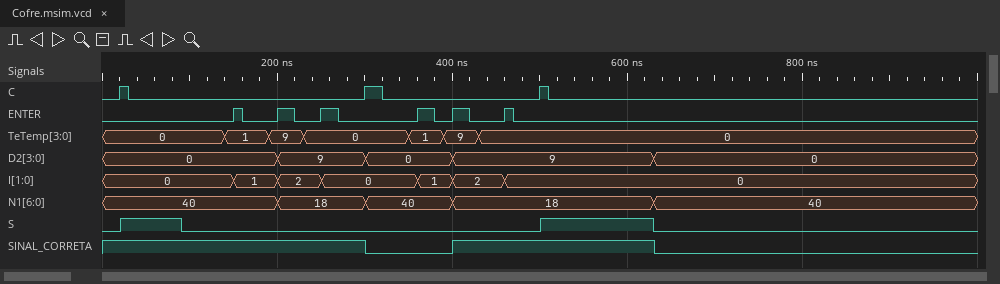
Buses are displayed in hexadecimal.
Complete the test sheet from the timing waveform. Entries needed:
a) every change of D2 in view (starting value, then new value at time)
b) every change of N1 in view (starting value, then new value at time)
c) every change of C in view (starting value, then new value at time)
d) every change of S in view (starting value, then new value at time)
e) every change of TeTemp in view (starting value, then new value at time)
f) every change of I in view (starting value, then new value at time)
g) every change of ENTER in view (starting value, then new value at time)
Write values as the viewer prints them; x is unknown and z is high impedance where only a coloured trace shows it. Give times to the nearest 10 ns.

0, 9 at 200 ns, 0 at 300 ns, 9 at 400 ns, 0 at 630 ns
40, 18 at 200 ns, 40 at 300 ns, 18 at 400 ns, 40 at 630 ns
0, 1 at 20 ns, 0 at 30 ns, 1 at 300 ns, 0 at 320 ns, 1 at 500 ns, 0 at 510 ns
0, 1 at 20 ns, 0 at 90 ns, 1 at 500 ns, 0 at 630 ns
0, 1 at 140 ns, 9 at 190 ns, 0 at 230 ns, 1 at 350 ns, 9 at 390 ns, 0 at 430 ns
0, 1 at 150 ns, 2 at 200 ns, 0 at 250 ns, 1 at 360 ns, 2 at 400 ns, 0 at 460 ns
0, 1 at 150 ns, 0 at 160 ns, 1 at 200 ns, 0 at 220 ns, 1 at 250 ns, 0 at 270 ns, 1 at 360 ns, 0 at 380 ns, 1 at 400 ns, 0 at 420 ns, 1 at 460 ns, 0 at 470 ns
